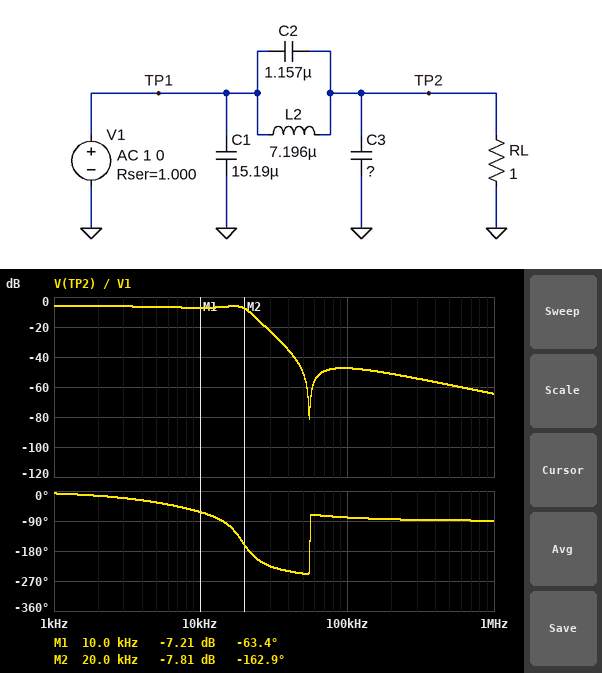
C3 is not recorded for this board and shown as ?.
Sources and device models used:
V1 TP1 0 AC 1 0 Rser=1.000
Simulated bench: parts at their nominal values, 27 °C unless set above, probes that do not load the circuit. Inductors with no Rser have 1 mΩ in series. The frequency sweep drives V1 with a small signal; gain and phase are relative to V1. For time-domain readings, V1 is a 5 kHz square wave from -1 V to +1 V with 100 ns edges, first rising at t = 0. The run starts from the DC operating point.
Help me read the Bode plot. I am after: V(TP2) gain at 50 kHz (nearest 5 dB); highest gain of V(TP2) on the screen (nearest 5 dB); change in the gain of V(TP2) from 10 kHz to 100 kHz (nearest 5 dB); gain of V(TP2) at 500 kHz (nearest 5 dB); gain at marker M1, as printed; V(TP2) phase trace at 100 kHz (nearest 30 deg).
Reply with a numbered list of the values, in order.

1. -50 dB
2. -5 dB
3. -40 dB
4. -60 dB
5. -7.21 dB
6. -90 deg
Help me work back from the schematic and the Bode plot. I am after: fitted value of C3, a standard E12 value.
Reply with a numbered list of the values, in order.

1. 18 µF
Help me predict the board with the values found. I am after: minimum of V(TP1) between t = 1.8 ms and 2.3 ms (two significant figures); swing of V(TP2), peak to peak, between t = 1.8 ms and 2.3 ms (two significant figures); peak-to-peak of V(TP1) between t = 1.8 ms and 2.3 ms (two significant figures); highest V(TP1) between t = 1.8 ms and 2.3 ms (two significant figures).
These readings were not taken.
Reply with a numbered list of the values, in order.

1. -570 mV
2. 1.1 V
3. 1.1 V
4. 570 mV
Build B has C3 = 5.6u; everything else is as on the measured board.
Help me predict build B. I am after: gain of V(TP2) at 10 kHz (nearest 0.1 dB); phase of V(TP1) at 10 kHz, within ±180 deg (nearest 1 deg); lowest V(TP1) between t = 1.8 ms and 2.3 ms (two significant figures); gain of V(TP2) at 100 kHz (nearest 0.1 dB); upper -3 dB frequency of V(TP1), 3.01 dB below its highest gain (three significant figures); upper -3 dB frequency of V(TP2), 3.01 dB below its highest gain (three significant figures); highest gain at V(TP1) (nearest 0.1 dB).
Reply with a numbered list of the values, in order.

1. -6.6 dB
2. -20 deg
3. -510 mV
4. -38.3 dB
5. 32.7 kHz
6. 23.7 kHz
7. -6.0 dB
